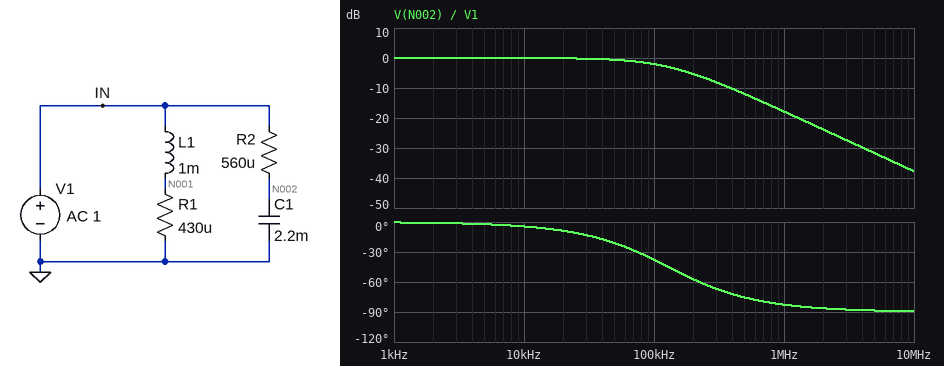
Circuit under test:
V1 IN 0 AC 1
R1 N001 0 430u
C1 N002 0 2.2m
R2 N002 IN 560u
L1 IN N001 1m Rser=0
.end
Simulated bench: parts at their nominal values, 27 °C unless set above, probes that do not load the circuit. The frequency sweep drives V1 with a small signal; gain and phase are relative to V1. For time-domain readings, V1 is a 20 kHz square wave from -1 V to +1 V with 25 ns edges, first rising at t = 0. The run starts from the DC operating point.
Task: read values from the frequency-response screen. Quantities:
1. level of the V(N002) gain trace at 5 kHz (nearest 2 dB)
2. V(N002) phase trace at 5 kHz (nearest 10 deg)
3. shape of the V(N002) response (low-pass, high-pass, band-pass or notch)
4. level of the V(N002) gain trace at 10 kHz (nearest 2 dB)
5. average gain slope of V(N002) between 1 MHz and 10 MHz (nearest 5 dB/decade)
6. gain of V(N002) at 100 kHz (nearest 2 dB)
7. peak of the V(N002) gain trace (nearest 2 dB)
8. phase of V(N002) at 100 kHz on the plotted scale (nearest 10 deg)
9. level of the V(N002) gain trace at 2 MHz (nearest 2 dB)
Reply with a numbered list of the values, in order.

1. 0 dB
2. 0 deg
3. low-pass
4. 0 dB
5. -20 dB/decade
6. -2 dB
7. 0 dB
8. -40 deg
9. -24 dB
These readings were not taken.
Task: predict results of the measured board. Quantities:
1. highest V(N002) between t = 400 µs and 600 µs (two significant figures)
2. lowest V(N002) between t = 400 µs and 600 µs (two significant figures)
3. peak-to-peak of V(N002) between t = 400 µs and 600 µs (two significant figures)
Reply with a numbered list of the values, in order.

1. 1.0 V
2. -1.0 V
3. 2.0 V
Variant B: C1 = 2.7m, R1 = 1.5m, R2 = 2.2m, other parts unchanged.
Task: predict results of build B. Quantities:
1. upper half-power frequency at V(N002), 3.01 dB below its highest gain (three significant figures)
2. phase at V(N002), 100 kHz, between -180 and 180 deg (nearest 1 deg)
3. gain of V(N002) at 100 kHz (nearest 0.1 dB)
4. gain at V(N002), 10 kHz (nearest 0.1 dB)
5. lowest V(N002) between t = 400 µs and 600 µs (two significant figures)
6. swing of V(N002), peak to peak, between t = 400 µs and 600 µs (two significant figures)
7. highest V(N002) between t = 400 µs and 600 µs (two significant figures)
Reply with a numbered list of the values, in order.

1. 26.8 kHz
2. -75 deg
3. -11.7 dB
4. -0.6 dB
5. -970 mV
6. 1.9 V
7. 970 mV
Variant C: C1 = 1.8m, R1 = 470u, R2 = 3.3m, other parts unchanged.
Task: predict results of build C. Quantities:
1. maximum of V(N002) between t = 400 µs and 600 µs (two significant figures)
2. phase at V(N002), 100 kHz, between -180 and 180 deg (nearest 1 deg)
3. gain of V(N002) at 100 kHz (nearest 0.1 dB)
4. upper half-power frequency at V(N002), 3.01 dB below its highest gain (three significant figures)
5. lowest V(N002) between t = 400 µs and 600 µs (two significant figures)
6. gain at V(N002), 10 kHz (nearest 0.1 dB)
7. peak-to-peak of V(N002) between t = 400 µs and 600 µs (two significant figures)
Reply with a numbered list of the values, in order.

1. 970 mV
2. -75 deg
3. -11.7 dB
4. 26.8 kHz
5. -970 mV
6. -0.6 dB
7. 1.9 V
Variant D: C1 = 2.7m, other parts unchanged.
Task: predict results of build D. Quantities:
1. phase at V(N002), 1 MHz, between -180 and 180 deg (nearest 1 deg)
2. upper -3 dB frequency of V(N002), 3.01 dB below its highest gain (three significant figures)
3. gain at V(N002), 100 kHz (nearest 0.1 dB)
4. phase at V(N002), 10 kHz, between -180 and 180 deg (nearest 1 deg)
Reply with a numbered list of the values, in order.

1. -84 deg
2. 105 kHz
3. -2.8 dB
4. -5 deg
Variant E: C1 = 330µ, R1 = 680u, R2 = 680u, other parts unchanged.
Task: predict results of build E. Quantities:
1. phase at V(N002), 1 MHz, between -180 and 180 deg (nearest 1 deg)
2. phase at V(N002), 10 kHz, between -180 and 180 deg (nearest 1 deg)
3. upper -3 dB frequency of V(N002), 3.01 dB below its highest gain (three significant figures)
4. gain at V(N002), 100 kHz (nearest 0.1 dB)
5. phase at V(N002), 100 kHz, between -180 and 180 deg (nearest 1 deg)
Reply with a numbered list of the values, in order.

1. -55 deg
2. -1 deg
3. 709 kHz
4. -0.1 dB
5. -8 deg
